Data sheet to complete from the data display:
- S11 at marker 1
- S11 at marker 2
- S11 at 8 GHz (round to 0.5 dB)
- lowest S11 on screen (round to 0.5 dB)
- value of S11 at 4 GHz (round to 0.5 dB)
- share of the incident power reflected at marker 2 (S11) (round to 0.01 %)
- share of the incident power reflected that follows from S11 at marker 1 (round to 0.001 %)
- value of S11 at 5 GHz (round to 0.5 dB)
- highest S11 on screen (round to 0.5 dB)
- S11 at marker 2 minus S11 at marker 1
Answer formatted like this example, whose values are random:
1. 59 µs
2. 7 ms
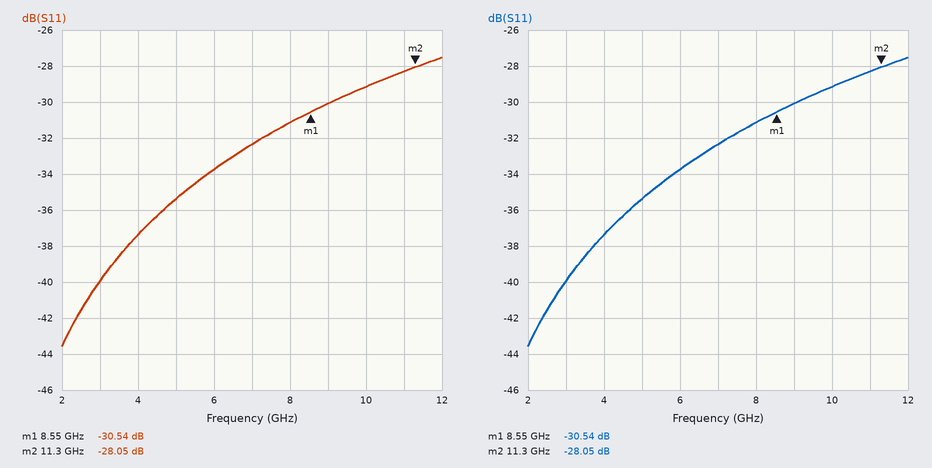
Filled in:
1. -30.54 dB
2. -28.05 dB
3. -31.0 dB
4. -43.5 dB
5. -37.5 dB
6. 0.16 %
7. 0.088 %
8. -35.5 dB
9. -27.5 dB
10. 2.49 dB
